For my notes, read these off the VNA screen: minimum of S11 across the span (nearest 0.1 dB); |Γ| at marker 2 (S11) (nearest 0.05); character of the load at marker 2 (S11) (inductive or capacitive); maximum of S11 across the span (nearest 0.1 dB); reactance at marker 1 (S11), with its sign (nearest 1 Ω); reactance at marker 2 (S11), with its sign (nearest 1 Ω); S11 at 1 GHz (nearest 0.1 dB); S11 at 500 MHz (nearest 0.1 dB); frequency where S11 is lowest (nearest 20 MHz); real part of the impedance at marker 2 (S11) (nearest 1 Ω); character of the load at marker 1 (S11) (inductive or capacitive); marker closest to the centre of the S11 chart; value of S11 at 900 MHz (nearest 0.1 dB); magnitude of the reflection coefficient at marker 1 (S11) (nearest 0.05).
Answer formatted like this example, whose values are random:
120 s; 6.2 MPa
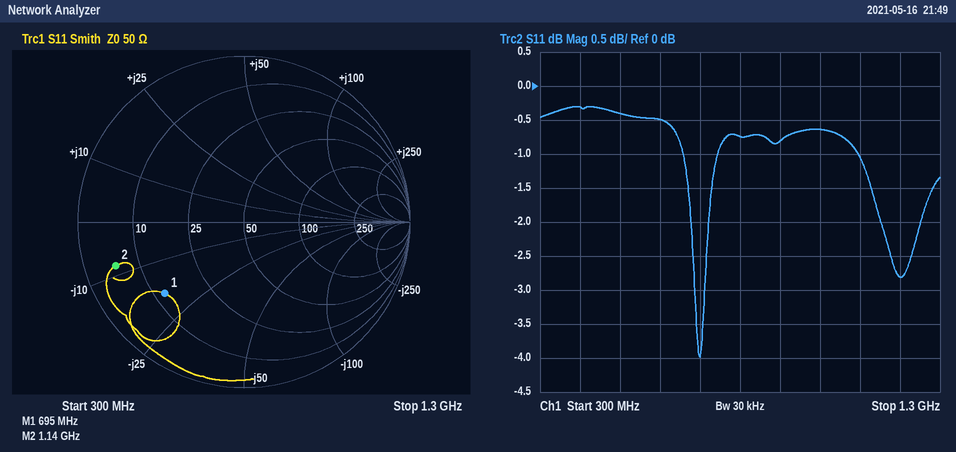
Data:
-4.0 dB; 0.80; capacitive; -0.3 dB; -18 Ω; -8 Ω; -0.6 dB; -0.4 dB; 700 MHz; 5 Ω; capacitive; marker 1; -0.8 dB; 0.65
